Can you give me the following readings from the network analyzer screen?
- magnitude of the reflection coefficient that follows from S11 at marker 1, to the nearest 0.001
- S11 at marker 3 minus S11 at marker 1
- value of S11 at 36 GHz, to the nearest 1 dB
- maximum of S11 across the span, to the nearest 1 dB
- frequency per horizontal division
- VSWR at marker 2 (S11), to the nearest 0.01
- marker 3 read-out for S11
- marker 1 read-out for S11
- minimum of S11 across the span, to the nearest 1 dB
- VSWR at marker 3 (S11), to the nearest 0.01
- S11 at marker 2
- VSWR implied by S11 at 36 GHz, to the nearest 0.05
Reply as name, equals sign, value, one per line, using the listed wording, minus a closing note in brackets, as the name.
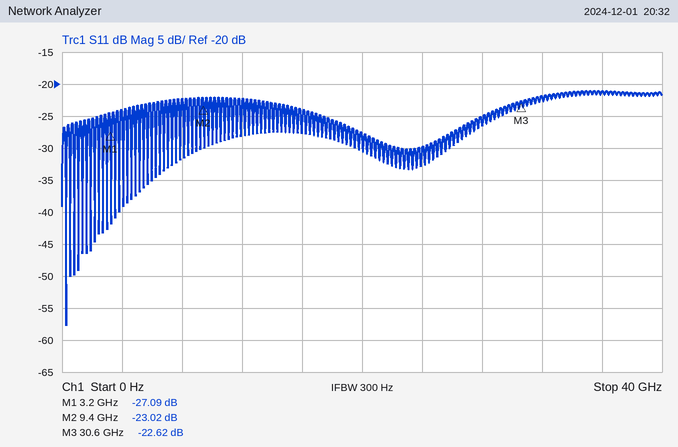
magnitude of the reflection coefficient that follows from S11 at marker 1, to the nearest 0.001 = 0.044
S11 at marker 3 minus S11 at marker 1 = 4.47 dB
value of S11 at 36 GHz, to the nearest 1 dB = -21 dB
maximum of S11 across the span, to the nearest 1 dB = -21 dB
frequency per horizontal division = 4 GHz
VSWR at marker 2 (S11), to the nearest 0.01 = 1.15
marker 3 read-out for S11 = -22.62 dB
marker 1 read-out for S11 = -27.09 dB
minimum of S11 across the span, to the nearest 1 dB = -58 dB
VSWR at marker 3 (S11), to the nearest 0.01 = 1.16
S11 at marker 2 = -23.02 dB
VSWR implied by S11 at 36 GHz, to the nearest 0.05 = 1.20
